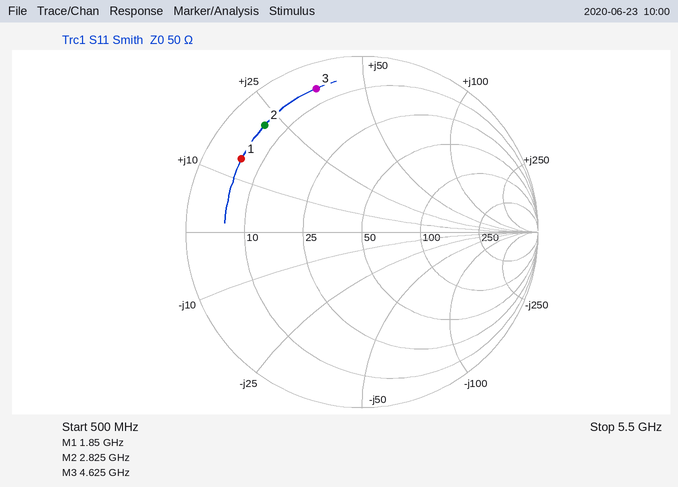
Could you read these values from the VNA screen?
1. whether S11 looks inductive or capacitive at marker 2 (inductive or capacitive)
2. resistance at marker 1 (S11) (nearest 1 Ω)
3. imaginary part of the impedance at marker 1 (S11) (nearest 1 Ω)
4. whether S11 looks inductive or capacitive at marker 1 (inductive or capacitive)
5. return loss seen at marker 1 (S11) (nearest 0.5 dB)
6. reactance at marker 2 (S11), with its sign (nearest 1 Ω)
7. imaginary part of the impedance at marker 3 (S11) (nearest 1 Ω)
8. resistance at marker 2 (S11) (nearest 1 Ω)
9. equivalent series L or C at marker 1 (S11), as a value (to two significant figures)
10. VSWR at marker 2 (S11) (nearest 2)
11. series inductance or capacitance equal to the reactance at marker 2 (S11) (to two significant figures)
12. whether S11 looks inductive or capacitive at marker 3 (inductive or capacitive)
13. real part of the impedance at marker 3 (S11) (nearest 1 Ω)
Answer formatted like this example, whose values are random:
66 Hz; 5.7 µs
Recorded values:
inductive; 6 Ω; +14 Ω; inductive; 2.0 dB; +22 Ω; +36 Ω; 6 Ω; 1.2 nH; 10; 1.2 nH; inductive; 6 Ω
